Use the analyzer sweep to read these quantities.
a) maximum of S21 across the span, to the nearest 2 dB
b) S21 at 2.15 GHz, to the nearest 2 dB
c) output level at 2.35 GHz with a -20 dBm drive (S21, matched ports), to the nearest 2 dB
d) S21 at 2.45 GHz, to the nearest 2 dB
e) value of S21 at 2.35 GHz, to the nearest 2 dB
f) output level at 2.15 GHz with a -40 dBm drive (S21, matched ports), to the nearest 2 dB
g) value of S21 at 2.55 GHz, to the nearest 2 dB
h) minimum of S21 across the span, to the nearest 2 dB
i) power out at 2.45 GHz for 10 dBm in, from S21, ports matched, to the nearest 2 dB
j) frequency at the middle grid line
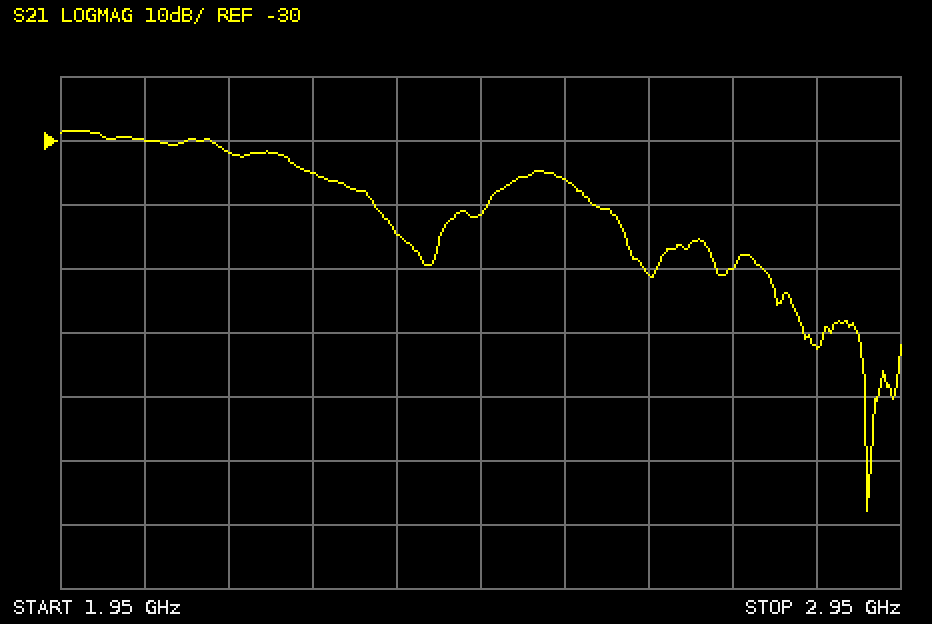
-28 dB
-32 dB
-64 dBm
-42 dB
-44 dB
-72 dBm
-36 dB
-88 dB
-32 dBm
2.45 GHz
